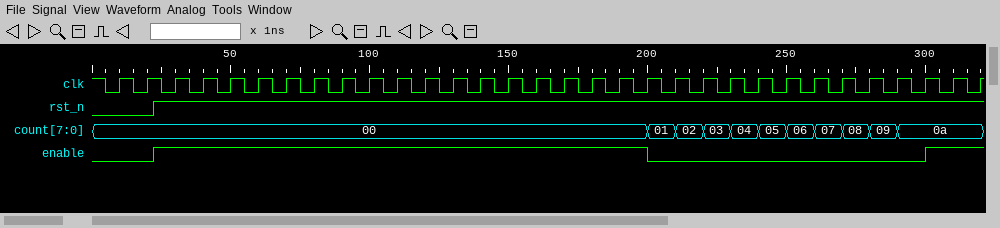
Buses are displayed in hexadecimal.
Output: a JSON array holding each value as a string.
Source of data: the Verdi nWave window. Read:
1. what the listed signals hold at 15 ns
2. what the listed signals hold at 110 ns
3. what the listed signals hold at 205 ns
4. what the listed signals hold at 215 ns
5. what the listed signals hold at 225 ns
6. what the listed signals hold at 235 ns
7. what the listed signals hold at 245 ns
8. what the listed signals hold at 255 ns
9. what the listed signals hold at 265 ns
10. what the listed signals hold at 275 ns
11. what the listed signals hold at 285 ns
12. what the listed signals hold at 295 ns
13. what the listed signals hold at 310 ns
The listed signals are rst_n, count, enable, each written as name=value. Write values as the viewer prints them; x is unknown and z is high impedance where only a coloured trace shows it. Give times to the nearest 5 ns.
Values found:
["rst_n=0, count=00, enable=0", "rst_n=1, count=00, enable=1", "rst_n=1, count=01, enable=0", "rst_n=1, count=02, enable=0", "rst_n=1, count=03, enable=0", "rst_n=1, count=04, enable=0", "rst_n=1, count=05, enable=0", "rst_n=1, count=06, enable=0", "rst_n=1, count=07, enable=0", "rst_n=1, count=08, enable=0", "rst_n=1, count=09, enable=0", "rst_n=1, count=0a, enable=0", "rst_n=1, count=0a, enable=1"]
